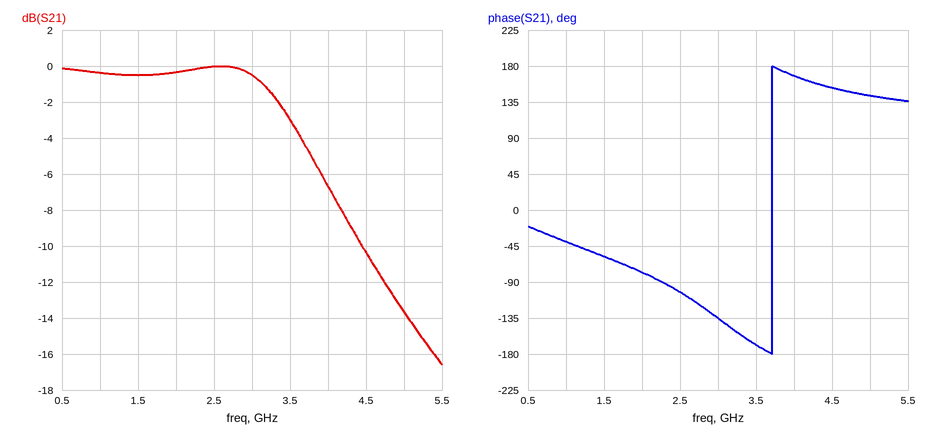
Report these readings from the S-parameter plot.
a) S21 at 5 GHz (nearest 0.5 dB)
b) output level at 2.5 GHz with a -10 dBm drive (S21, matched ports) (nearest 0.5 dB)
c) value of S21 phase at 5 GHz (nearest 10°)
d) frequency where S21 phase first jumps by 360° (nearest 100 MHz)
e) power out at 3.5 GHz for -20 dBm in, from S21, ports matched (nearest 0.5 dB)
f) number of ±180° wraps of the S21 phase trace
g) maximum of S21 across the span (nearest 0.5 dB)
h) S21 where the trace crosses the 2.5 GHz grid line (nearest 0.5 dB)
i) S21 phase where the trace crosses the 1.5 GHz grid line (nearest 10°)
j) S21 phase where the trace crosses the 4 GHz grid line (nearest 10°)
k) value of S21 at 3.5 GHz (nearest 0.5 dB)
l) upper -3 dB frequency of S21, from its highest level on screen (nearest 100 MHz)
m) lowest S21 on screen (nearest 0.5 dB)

-13.5 dB
-10.0 dBm
140°
3.7 GHz
-23.0 dBm
1
0.0 dB
0.0 dB
-60°
170°
-3.0 dB
3.5 GHz
-16.5 dB
